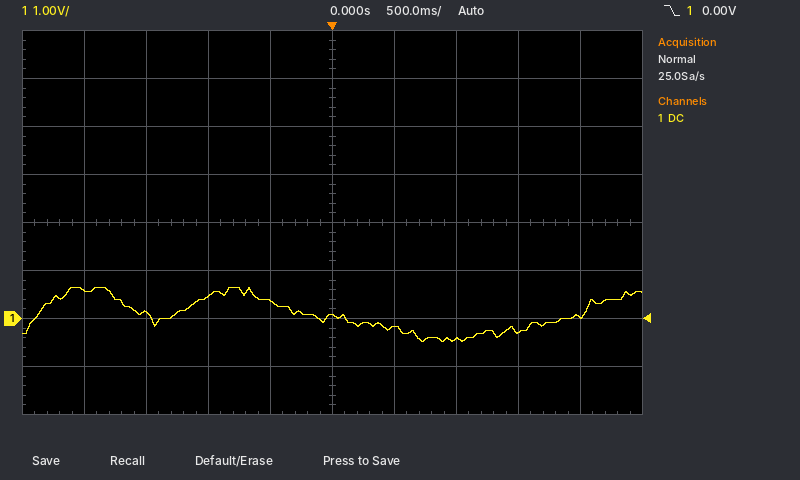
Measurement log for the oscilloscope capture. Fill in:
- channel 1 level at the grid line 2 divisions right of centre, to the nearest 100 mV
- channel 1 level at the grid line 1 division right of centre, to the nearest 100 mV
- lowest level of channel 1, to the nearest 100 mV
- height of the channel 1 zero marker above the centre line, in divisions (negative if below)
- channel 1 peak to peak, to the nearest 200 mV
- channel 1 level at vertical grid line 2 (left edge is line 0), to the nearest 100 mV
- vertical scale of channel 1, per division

-400 mV
-200 mV
-500 mV
-2.0 div
1.2 V
100 mV
1 V
